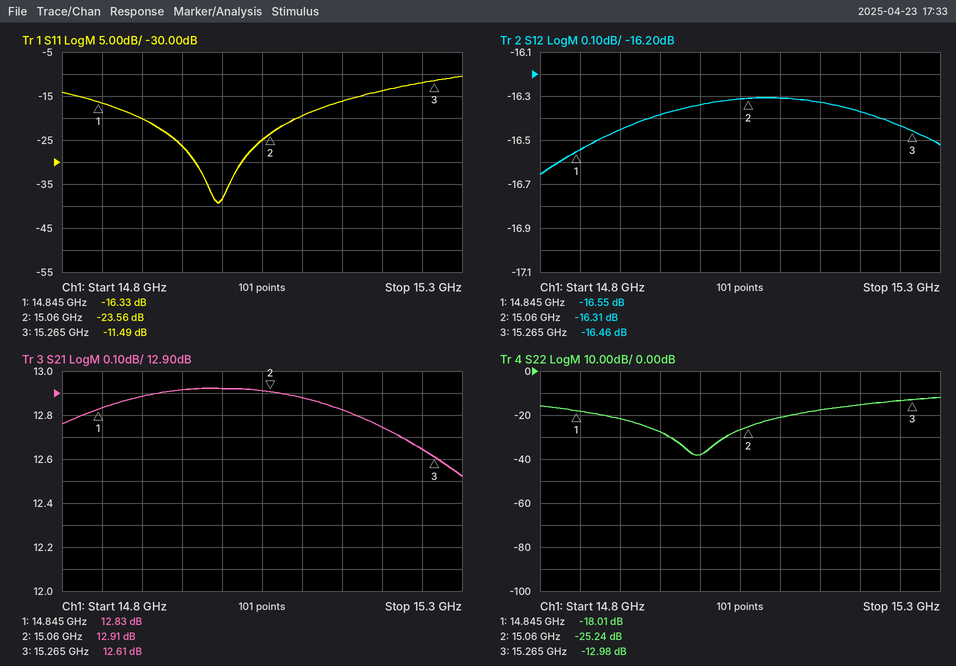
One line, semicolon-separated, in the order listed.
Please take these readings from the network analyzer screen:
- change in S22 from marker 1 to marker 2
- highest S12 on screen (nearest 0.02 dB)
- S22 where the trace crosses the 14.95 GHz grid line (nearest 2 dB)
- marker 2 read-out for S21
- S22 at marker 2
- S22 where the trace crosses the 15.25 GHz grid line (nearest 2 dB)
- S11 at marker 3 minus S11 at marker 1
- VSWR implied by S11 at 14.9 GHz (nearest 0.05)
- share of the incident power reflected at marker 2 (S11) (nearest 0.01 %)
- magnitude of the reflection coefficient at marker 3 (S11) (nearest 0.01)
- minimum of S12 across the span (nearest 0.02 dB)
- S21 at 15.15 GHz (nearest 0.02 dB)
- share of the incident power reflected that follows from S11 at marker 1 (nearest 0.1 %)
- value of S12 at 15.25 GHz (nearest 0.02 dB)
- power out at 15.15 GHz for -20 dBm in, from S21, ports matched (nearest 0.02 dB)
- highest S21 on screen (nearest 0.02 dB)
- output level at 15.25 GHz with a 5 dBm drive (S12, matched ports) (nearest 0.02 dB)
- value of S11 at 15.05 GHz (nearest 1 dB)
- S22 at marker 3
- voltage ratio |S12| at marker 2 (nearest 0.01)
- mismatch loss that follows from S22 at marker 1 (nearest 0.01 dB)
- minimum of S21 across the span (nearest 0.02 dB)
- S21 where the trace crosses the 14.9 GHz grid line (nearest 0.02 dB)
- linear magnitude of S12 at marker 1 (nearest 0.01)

-7.23 dB; -16.30 dB; -28 dB; 12.91 dB; -25.24 dB; -14 dB; 4.84 dB; 1.20; 0.44 %; 0.27; -16.66 dB; 12.82 dB; 2.3 %; -16.44 dB; -7.18 dBm; 12.92 dB; -11.44 dBm; -25 dB; -12.98 dB; 0.15; 0.07 dB; 12.52 dB; 12.88 dB; 0.15
